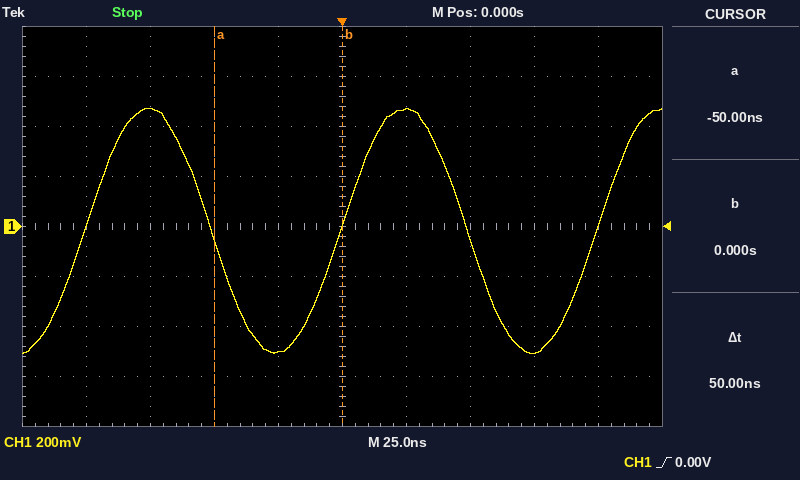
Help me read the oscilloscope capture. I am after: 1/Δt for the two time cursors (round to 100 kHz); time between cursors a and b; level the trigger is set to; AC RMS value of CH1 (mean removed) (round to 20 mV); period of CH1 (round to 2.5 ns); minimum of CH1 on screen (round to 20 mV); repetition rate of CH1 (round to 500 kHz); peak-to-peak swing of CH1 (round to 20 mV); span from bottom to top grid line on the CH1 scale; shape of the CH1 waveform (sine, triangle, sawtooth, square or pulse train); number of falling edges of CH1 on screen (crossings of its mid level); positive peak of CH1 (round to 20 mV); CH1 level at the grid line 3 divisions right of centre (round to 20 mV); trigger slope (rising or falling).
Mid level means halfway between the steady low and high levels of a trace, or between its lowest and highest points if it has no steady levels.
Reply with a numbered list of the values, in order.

1. 20.0 MHz
2. 50 ns
3. 0.00 V
4. 340 mV
5. 100.0 ns
6. -500 mV
7. 10.0 MHz
8. 980 mV
9. 1.6 V
10. sine
11. 2
12. 480 mV
13. -500 mV
14. rising
